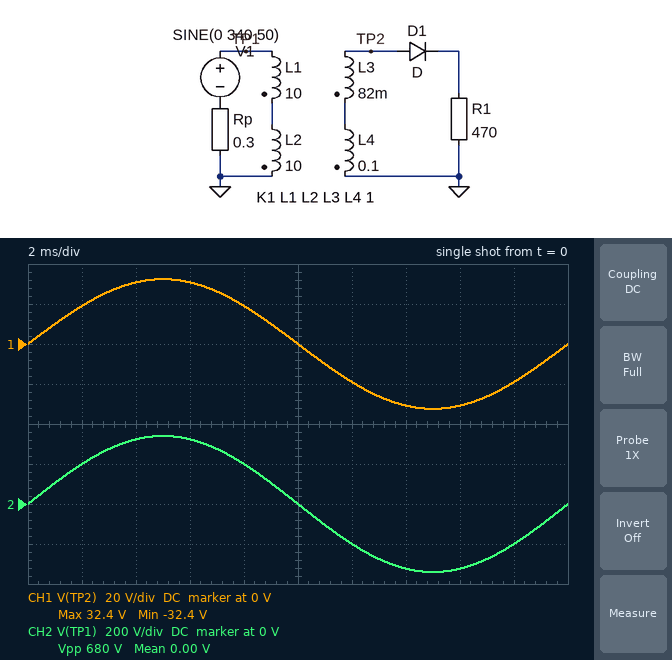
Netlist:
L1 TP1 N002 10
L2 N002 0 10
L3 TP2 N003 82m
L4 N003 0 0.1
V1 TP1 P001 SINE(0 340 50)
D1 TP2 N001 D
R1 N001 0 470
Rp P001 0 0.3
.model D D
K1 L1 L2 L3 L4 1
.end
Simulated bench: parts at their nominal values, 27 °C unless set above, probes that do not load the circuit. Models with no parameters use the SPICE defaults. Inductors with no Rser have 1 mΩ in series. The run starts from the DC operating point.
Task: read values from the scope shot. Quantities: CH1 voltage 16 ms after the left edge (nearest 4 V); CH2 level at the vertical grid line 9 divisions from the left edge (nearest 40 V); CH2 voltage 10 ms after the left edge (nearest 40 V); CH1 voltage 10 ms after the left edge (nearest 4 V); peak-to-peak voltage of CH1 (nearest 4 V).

-32 V
-200 V
0 V
0 V
64 V
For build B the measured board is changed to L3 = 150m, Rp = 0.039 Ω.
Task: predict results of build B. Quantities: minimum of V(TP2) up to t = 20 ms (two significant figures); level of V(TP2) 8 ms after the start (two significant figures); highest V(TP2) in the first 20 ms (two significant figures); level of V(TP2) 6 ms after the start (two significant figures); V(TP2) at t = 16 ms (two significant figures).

-38 V
22 V
38 V
36 V
-36 V
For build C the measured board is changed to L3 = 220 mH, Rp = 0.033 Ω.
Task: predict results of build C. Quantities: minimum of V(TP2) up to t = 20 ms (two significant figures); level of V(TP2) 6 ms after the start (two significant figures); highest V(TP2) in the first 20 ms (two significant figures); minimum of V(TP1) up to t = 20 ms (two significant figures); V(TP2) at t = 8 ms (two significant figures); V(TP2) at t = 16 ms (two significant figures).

-42 V
40 V
42 V
-340 V
25 V
-40 V
